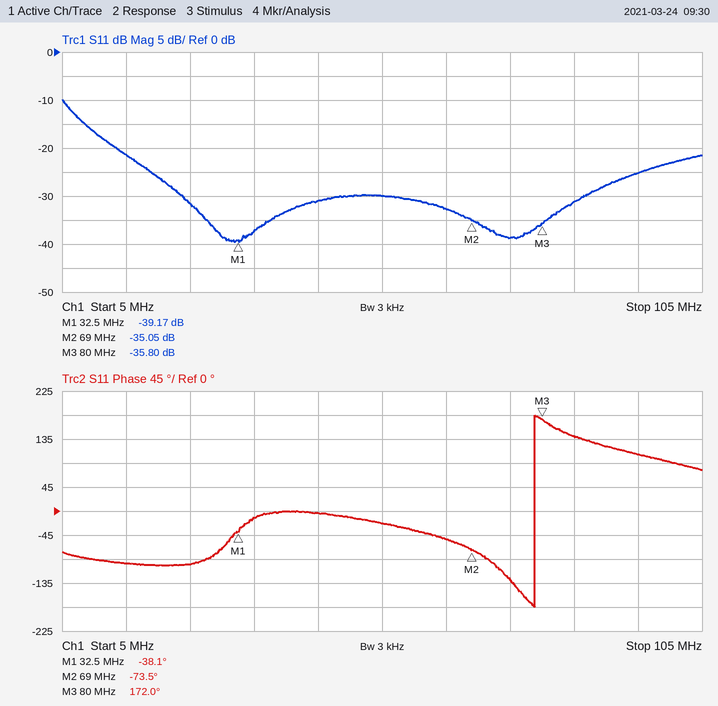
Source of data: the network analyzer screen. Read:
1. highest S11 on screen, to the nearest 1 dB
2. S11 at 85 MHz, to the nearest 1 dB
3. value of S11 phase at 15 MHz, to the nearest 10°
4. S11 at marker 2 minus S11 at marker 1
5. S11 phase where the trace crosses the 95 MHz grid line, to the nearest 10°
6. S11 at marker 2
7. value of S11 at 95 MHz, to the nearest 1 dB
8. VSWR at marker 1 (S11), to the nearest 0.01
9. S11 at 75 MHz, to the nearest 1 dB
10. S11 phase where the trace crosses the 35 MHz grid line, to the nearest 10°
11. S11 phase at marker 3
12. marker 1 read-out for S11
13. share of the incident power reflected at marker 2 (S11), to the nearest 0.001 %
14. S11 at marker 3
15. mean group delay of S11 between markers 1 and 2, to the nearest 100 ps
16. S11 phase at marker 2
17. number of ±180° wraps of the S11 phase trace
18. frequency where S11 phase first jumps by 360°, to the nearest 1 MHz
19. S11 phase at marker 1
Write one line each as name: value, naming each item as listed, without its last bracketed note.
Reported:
highest S11 on screen, to the nearest 1 dB: -10 dB
S11 at 85 MHz, to the nearest 1 dB: -31 dB
value of S11 phase at 15 MHz, to the nearest 10°: -100°
S11 at marker 2 minus S11 at marker 1: 4.12 dB
S11 phase where the trace crosses the 95 MHz grid line, to the nearest 10°: 110°
S11 at marker 2: -35.05 dB
value of S11 at 95 MHz, to the nearest 1 dB: -25 dB
VSWR at marker 1 (S11), to the nearest 0.01: 1.02
S11 at 75 MHz, to the nearest 1 dB: -39 dB
S11 phase where the trace crosses the 35 MHz grid line, to the nearest 10°: -10°
S11 phase at marker 3: 172.0°
marker 1 read-out for S11: -39.17 dB
share of the incident power reflected at marker 2 (S11), to the nearest 0.001 %: 0.031 %
S11 at marker 3: -35.80 dB
mean group delay of S11 between markers 1 and 2, to the nearest 100 ps: 2.7 ns
S11 phase at marker 2: -73.5°
number of ±180° wraps of the S11 phase trace: 1
frequency where S11 phase first jumps by 360°, to the nearest 1 MHz: 79 MHz
S11 phase at marker 1: -38.1°
